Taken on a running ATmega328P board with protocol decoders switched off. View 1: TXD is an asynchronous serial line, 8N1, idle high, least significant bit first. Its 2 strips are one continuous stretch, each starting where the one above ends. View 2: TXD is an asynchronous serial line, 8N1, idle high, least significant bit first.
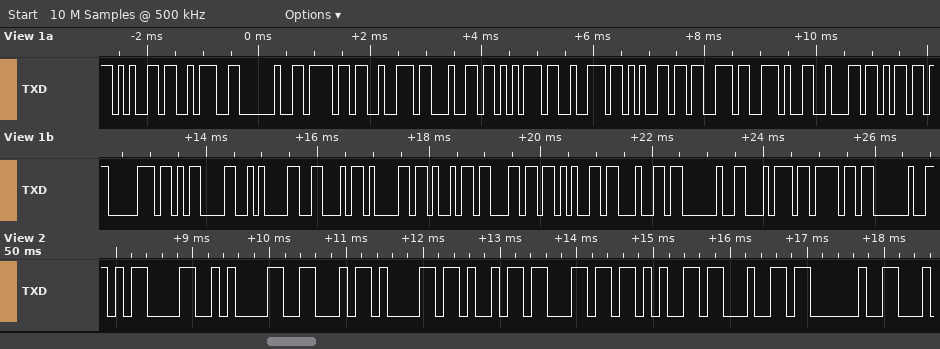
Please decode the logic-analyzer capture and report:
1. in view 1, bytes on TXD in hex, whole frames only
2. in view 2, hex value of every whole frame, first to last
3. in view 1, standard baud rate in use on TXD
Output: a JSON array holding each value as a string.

["65 3A 20 6F 72 64 75 72 65 73 2E 62 6D 70 0D 0A 46 61 69 6C 65 64 20 74 6F 20", "0D 0A 46 61 69 6C 65 64 20", "9600 baud"]
